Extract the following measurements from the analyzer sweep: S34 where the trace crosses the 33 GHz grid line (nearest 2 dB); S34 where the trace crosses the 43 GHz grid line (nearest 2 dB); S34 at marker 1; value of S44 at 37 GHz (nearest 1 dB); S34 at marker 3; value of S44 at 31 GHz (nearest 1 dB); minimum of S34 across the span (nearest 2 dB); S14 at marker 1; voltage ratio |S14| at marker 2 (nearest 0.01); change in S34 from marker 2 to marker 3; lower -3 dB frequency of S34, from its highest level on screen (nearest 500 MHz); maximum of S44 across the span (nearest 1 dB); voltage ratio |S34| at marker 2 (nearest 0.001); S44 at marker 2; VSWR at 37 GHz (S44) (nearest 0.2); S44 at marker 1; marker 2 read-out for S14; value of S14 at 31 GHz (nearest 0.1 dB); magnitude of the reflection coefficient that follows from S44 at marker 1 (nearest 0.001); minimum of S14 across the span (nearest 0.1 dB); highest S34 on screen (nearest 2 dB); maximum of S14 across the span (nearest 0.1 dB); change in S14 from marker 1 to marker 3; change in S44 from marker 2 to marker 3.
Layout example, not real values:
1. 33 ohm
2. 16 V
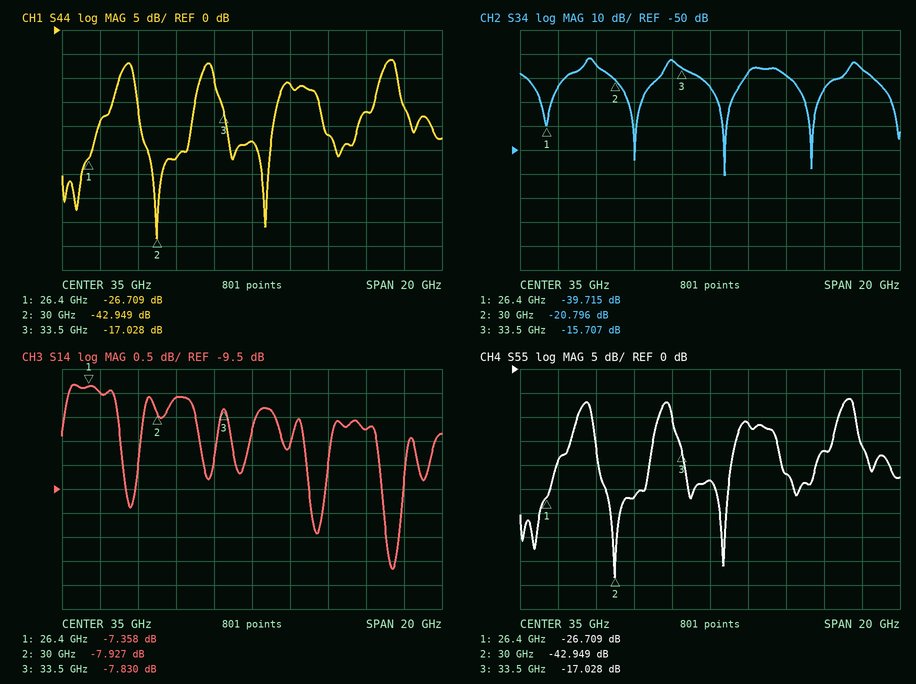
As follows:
1. -12 dB
2. -16 dB
3. -39.715 dB
4. -11 dB
5. -15.707 dB
6. -27 dB
7. -60 dB
8. -7.358 dB
9. 0.40
10. 5.089 dB
11. 28.5 GHz
12. -6 dB
13. 0.091
14. -42.949 dB
15. 1.8
16. -26.709 dB
17. -7.927 dB
18. -7.6 dB
19. 0.046
20. -11.2 dB
21. -12 dB
22. -7.3 dB
23. -0.472 dB
24. 25.921 dB
